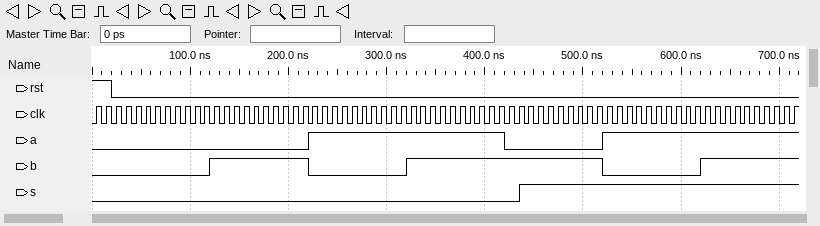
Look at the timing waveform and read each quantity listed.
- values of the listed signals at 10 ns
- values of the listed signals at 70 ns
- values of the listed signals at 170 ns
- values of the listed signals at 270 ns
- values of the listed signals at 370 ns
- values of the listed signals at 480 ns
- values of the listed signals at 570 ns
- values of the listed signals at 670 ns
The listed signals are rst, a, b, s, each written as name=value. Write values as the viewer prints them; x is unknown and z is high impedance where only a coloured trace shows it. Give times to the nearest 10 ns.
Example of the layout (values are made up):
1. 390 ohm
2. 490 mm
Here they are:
1. rst=1, a=0, b=0, s=0
2. rst=0, a=0, b=0, s=0
3. rst=0, a=0, b=1, s=0
4. rst=0, a=1, b=0, s=0
5. rst=0, a=1, b=1, s=0
6. rst=0, a=0, b=1, s=1
7. rst=0, a=1, b=0, s=1
8. rst=0, a=1, b=1, s=1
